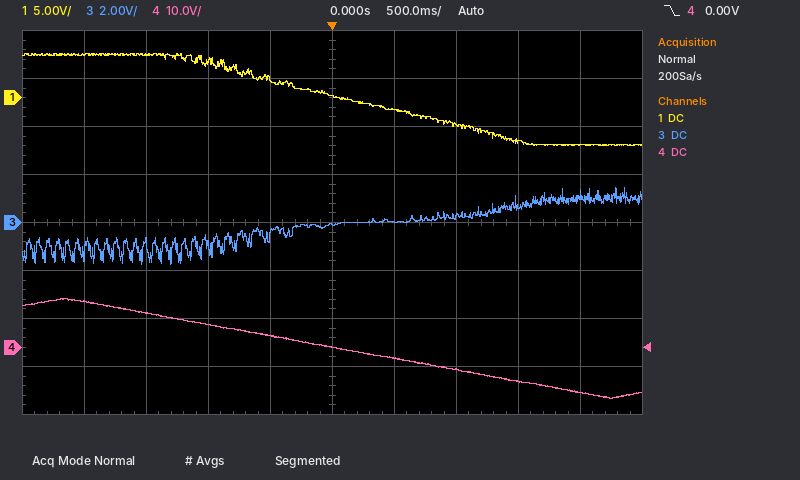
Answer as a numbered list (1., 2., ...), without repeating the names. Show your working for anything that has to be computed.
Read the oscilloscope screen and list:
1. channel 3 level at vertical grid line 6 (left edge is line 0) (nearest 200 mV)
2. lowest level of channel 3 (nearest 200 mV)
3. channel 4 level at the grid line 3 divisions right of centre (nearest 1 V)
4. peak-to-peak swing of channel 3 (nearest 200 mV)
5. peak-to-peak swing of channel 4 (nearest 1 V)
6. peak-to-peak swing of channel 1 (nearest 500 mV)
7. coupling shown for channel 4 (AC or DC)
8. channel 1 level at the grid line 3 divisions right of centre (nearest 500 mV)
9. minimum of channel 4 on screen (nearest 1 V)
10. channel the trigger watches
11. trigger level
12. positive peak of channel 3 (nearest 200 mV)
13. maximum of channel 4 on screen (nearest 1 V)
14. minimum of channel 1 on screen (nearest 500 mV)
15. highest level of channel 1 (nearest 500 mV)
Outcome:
1. 0.0 V
2. -1.8 V
3. -7 V
4. 1.4 V − (-1.8 V) = 3.2 V
5. 10 V − (-11 V) = 21 V
6. 4.5 V − (-5.0 V) = 9.5 V
7. DC
8. -4.5 V
9. -11 V
10. channel 4
11. 0.00 V
12. 1.4 V
13. 10 V
14. -5.0 V
15. 4.5 V
